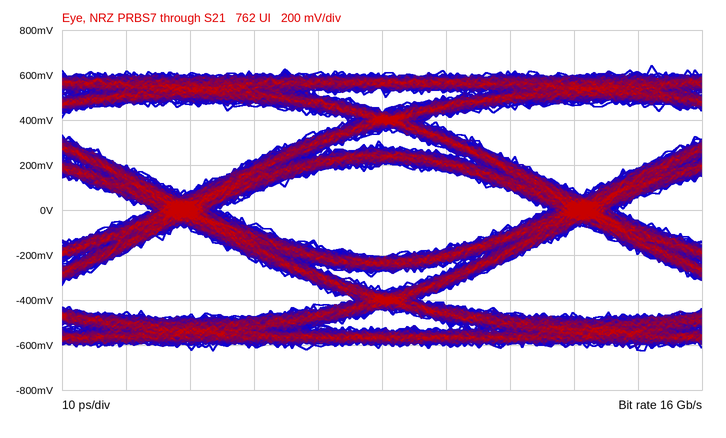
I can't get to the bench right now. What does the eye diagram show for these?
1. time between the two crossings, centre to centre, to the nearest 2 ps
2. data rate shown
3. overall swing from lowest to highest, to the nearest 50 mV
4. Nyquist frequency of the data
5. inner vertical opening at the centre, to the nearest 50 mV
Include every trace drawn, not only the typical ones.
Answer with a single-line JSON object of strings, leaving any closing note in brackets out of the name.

{"time between the two crossings, centre to centre, to the nearest 2 ps": "62 ps", "data rate shown": "16 Gb/s", "overall swing from lowest to highest, to the nearest 50 mV": "1.25 V", "Nyquist frequency of the data": "8 GHz", "inner vertical opening at the centre, to the nearest 50 mV": "400 mV"}
